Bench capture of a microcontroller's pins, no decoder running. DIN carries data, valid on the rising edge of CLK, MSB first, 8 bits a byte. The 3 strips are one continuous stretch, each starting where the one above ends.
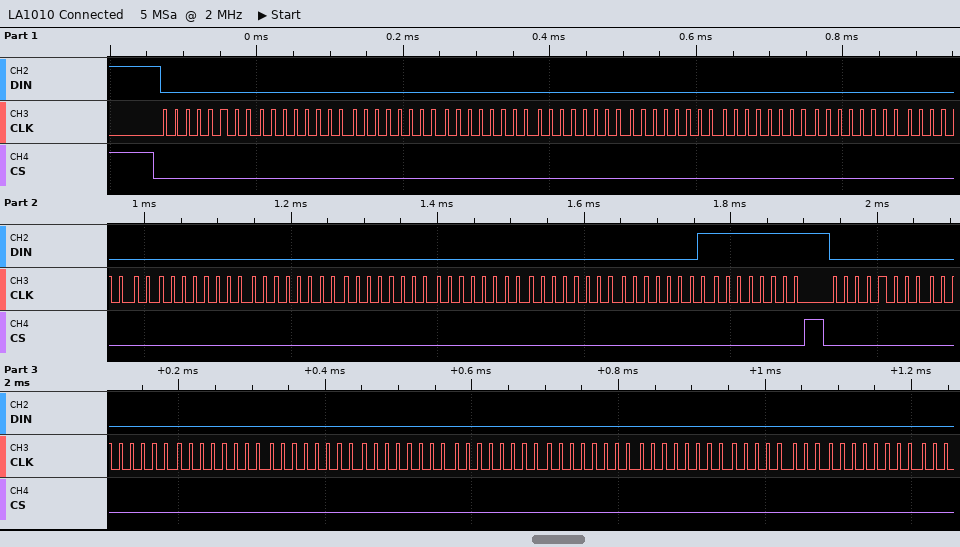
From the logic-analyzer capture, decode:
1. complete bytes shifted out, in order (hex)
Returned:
00 00 00 00 00 00 00 00 00 00 00 00 00 00 01 FF 00 00 00 00 00 00 00 00 00 00
